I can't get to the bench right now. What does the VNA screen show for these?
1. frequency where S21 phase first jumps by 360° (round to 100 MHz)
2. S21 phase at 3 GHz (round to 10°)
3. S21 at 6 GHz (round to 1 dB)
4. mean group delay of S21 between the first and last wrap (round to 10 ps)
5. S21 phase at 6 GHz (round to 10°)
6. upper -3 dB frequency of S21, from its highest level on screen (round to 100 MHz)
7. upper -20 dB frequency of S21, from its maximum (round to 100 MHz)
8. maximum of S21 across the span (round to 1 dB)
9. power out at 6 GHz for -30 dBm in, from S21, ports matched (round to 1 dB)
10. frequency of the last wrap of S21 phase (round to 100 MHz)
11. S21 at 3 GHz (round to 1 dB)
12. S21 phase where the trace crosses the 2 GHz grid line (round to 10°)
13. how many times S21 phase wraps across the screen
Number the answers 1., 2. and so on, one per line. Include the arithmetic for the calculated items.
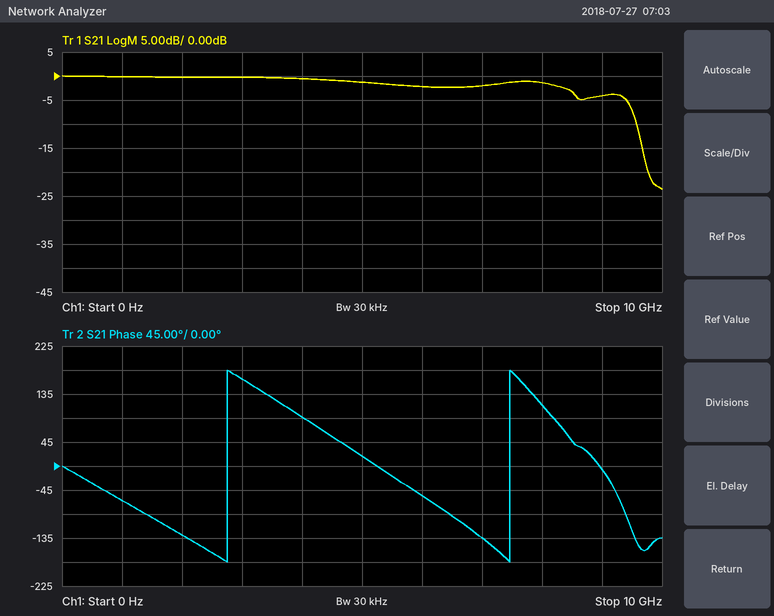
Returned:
1. 2.8 GHz
2. 160°
3. -2 dB
4. 1 cycle / (7.5 GHz − 2.8 GHz) ≈ 213 ps, so 210 ps to the nearest 10 ps
5. -60°
6. 8.5 GHz
7. 9.8 GHz
8. 0 dB
9. -30 dBm + (-2 dB) = -32 dBm
10. 7.5 GHz
11. 0 dB
12. -130°
13. 2
